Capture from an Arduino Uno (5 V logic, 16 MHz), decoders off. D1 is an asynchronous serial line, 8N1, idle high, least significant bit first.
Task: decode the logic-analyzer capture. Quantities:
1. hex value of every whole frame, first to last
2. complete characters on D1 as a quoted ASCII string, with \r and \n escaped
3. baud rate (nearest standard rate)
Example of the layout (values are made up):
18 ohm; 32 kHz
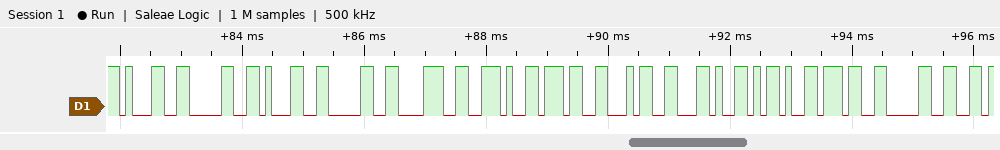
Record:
0x31 0x30 0x31 0x30 0x38 0x2E 0x37 0x34 0x2C 0x2D 0x37 0x30; "10108.74,-70"; 9600 baud
